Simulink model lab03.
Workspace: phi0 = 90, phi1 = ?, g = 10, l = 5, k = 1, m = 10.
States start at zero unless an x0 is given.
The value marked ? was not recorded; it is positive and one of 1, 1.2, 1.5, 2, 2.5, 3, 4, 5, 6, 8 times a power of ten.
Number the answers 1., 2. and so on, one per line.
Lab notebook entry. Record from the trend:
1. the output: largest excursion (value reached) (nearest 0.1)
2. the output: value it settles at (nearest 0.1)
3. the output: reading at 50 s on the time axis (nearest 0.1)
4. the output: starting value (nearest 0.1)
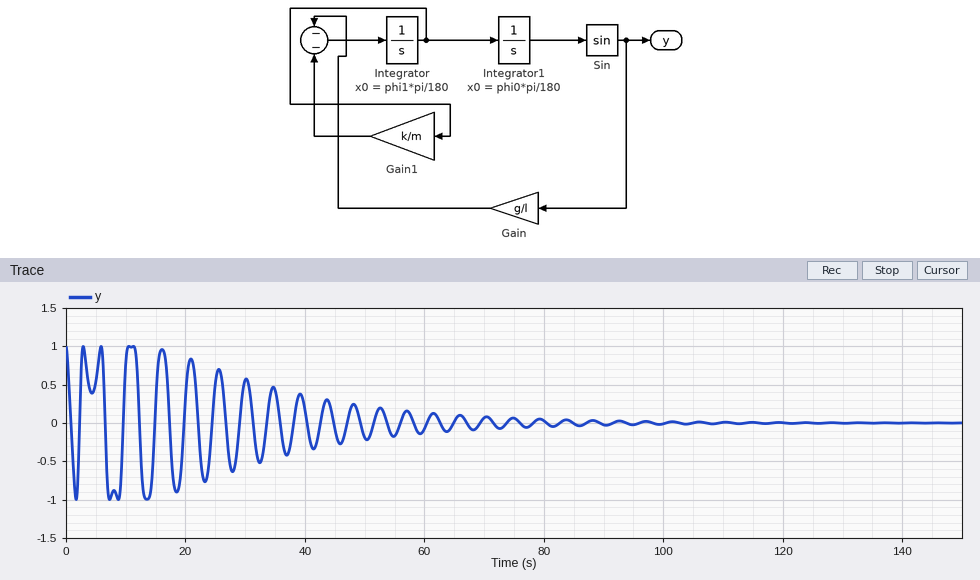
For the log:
1. -1.0
2. 0.0
3. -0.2
4. 1.0
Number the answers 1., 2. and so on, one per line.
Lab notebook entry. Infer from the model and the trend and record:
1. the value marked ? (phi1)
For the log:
1. 150
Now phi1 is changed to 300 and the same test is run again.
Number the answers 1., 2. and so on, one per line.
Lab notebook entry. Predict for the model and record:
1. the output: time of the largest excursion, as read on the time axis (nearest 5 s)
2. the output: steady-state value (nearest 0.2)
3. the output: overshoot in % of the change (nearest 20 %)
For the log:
1. 20 s
2. 0.0
3. 100 %
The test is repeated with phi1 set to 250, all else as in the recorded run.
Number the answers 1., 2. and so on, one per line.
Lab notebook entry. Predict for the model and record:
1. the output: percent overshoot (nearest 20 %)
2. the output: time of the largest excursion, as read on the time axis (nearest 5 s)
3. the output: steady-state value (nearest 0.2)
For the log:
1. 100 %
2. 15 s
3. 0.0
